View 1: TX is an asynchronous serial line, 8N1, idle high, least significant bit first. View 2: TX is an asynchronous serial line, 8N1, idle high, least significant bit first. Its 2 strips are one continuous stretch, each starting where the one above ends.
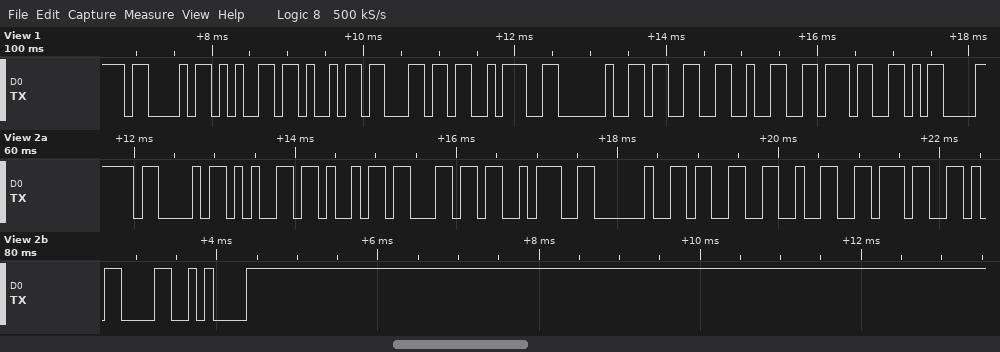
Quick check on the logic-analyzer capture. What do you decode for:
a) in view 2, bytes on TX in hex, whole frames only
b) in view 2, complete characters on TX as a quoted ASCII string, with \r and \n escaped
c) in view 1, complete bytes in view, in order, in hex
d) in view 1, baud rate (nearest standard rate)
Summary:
43 65 69 6C 3A 20 33 32 37 0D 0A
"Ceil: 327\r\n"
0x43 0x65 0x69 0x6C 0x3A 0x20 0x33 0x32 0x37 0x0D
9600 baud
